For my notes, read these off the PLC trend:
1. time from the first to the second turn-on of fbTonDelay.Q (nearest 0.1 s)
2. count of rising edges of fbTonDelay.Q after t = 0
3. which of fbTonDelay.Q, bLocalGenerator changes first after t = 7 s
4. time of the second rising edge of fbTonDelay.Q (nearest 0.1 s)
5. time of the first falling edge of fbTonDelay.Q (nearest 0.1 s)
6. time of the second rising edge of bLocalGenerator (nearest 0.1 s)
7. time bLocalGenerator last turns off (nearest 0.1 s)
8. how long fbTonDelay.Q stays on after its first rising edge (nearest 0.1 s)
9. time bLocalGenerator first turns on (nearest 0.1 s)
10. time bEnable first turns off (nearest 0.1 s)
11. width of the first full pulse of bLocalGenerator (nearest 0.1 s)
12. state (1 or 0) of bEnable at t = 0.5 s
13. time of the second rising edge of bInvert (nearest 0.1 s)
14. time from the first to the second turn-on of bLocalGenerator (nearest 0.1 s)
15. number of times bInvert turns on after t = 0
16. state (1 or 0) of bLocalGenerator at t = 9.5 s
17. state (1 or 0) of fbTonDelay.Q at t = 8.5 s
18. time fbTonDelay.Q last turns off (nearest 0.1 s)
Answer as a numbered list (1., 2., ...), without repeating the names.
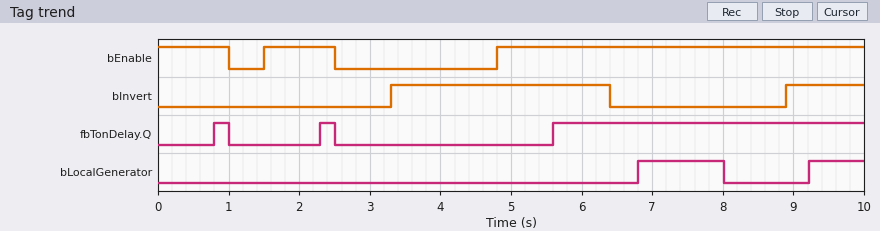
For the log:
1. 1.5 s
2. 3
3. bLocalGenerator
4. 2.3 s
5. 1.0 s
6. 9.2 s
7. 8.0 s
8. 0.2 s
9. 6.8 s
10. 1.0 s
11. 1.2 s
12. 1
13. 8.9 s
14. 2.4 s
15. 2
16. 1
17. 1
18. 2.5 s
